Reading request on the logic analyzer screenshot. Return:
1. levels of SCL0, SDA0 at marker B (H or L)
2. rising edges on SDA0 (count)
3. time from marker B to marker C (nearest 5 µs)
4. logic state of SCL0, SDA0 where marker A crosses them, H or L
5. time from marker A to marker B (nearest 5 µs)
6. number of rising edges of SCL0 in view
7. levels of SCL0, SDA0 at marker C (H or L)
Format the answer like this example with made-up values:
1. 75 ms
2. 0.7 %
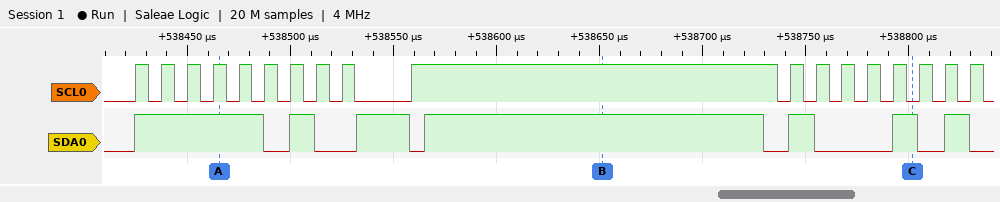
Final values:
1. SCL0=H, SDA0=H
2. 7
3. 150 µs
4. SCL0=H, SDA0=H
5. 185 µs
6. 18
7. SCL0=L, SDA0=H
